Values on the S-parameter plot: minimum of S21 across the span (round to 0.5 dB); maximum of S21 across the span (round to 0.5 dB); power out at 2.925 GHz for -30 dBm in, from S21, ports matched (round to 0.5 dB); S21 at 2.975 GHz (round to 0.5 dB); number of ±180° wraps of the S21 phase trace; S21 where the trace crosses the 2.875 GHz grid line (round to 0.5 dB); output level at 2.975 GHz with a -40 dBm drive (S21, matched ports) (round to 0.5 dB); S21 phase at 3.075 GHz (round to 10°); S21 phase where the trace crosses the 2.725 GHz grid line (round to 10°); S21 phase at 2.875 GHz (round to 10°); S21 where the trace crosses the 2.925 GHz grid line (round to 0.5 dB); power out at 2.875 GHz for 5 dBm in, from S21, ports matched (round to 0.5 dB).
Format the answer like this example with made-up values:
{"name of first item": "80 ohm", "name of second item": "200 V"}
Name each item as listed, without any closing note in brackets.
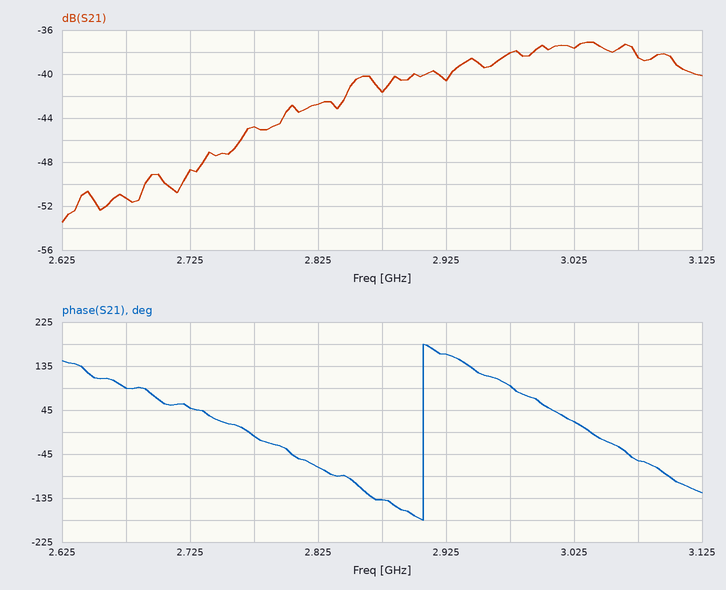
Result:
{"minimum of S21 across the span": "-53.5 dB", "maximum of S21 across the span": "-37.0 dB", "power out at 2.925 GHz for -30 dBm in, from S21, ports matched": "-70.5 dBm", "S21 at 2.975 GHz": "-38.0 dB", "number of ±180° wraps of the S21 phase trace": "1", "S21 where the trace crosses the 2.875 GHz grid line": "-41.5 dB", "output level at 2.975 GHz with a -40 dBm drive (S21, matched ports)": "-78.0 dBm", "S21 phase at 3.075 GHz": "-60°", "S21 phase where the trace crosses the 2.725 GHz grid line": "50°", "S21 phase at 2.875 GHz": "-140°", "S21 where the trace crosses the 2.925 GHz grid line": "-40.5 dB", "power out at 2.875 GHz for 5 dBm in, from S21, ports matched": "-36.5 dBm"}
